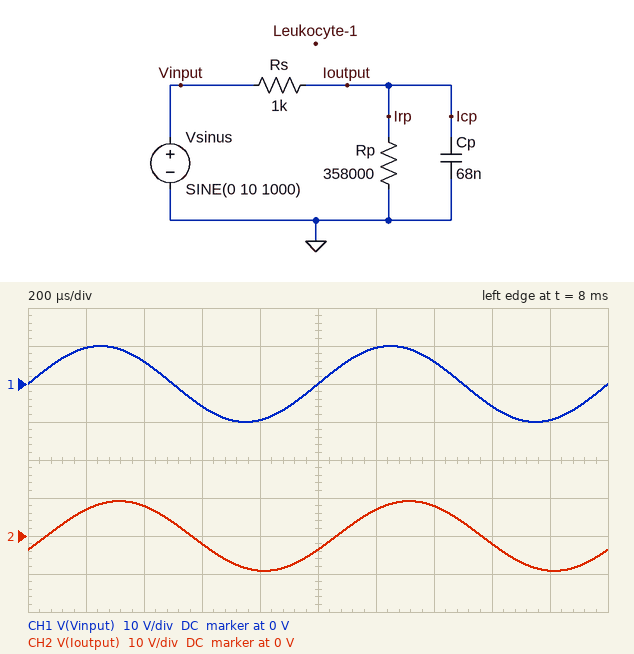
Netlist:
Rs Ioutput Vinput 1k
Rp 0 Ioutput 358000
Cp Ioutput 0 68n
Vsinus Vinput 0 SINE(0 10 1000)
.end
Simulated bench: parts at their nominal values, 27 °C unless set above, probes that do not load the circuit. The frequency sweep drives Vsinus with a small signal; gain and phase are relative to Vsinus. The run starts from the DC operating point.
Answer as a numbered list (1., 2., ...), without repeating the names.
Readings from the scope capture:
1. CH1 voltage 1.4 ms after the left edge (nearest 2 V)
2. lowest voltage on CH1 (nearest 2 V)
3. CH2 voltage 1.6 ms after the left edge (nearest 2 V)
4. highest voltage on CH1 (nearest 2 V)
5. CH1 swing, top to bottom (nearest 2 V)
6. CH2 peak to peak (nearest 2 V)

1. 6 V
2. -10 V
3. -2 V
4. 10 V
5. 20 V
6. 18 V
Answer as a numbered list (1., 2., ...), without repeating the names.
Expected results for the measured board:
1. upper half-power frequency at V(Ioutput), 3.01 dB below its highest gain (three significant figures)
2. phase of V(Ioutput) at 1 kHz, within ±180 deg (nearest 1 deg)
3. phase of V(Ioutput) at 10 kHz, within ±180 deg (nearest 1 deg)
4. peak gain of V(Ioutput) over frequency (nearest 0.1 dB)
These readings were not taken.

1. 2.35 kHz
2. -23 deg
3. -77 deg
4. 0 dB
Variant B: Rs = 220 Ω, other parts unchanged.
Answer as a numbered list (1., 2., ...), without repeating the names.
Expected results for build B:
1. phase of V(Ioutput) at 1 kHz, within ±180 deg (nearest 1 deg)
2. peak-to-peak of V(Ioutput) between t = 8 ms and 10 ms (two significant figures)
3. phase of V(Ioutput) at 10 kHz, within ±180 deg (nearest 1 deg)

1. -5 deg
2. 20 V
3. -43 deg
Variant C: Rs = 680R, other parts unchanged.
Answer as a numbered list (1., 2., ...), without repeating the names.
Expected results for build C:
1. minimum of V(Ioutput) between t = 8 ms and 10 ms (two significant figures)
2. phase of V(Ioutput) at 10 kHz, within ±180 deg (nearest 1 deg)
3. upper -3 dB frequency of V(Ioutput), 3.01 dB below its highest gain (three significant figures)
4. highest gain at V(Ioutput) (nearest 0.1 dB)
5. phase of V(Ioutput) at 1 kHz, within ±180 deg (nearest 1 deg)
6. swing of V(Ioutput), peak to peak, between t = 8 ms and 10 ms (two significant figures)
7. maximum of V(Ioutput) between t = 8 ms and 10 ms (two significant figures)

1. -9.6 V
2. -71 deg
3. 3.45 kHz
4. 0 dB
5. -16 deg
6. 19 V
7. 9.6 V
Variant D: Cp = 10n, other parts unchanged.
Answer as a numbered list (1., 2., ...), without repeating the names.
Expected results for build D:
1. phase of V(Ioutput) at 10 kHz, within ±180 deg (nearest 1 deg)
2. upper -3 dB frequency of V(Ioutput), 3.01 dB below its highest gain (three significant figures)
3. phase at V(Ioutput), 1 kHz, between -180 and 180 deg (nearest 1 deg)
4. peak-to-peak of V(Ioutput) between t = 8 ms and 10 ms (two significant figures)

1. -32 deg
2. 16.0 kHz
3. -4 deg
4. 20 V
